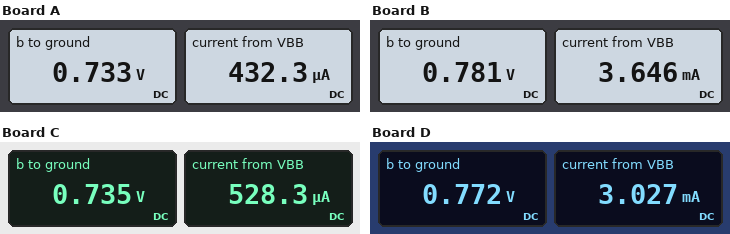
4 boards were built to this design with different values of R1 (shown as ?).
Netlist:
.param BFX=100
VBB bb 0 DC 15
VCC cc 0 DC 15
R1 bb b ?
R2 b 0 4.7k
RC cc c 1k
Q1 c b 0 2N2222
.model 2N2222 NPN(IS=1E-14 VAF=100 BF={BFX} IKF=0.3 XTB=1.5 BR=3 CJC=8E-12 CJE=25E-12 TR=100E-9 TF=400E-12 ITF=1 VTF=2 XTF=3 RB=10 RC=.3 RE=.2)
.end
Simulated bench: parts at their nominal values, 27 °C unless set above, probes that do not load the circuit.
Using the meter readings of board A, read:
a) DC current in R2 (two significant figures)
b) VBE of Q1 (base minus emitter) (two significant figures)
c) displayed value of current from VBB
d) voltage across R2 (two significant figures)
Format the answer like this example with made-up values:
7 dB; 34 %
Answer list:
160 µA; 730 mV; 432.3 µA; 730 mV
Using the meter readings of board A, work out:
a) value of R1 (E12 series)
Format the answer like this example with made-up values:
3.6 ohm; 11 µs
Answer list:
33 kΩ
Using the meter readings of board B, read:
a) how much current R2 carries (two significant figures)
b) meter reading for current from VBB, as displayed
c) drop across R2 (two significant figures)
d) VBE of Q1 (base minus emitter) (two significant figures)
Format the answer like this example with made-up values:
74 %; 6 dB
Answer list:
170 µA; 3.646 mA; 780 mV; 780 mV
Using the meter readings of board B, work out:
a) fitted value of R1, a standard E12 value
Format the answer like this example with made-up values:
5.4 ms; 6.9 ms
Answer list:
3.9 kΩ
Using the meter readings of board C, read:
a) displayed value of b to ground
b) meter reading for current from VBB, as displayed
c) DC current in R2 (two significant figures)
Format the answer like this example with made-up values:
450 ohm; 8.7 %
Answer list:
0.735 V; 528.3 µA; 160 µA
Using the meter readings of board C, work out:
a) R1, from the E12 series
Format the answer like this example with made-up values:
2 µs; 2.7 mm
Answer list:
27 kΩ
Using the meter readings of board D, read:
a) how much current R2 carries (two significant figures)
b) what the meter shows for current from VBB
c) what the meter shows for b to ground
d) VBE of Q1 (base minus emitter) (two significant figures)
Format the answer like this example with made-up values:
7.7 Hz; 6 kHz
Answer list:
160 µA; 3.027 mA; 0.772 V; 770 mV
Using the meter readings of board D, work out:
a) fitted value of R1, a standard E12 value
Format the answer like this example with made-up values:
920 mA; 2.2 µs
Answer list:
4.7 kΩ
